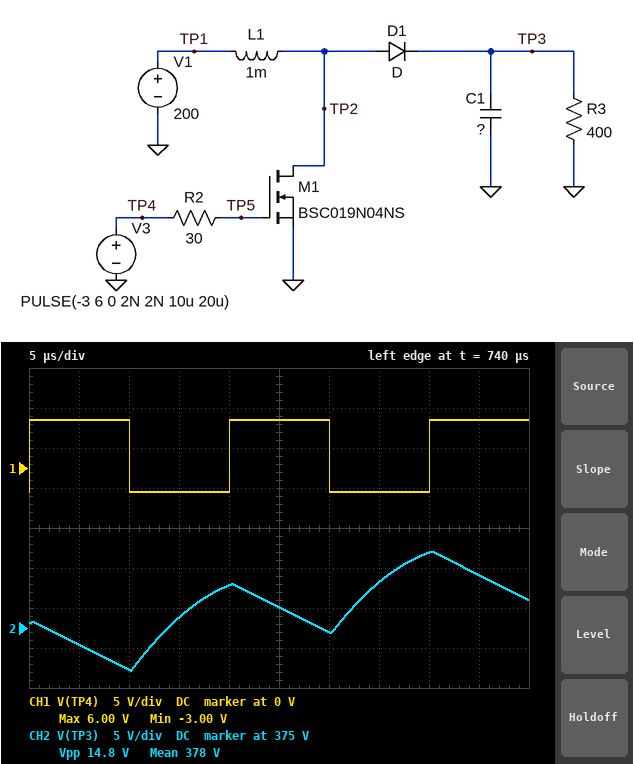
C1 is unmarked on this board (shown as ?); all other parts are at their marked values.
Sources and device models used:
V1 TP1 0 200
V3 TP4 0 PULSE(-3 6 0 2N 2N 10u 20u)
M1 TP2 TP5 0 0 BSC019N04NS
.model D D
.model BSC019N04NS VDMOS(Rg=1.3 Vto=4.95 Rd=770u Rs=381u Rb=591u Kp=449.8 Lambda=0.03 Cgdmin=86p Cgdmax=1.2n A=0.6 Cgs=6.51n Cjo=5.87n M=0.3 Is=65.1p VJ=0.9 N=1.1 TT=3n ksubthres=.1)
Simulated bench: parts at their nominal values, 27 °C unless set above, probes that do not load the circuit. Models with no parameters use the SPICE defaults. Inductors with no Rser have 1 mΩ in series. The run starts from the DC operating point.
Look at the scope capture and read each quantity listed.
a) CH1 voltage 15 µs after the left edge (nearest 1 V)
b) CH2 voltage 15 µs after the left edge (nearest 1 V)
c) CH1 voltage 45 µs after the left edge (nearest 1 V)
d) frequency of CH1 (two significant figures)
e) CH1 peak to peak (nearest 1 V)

-3 V
376 V
6 V
50 kHz
9 V
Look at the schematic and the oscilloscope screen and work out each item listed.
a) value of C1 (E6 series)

1.5 µF
